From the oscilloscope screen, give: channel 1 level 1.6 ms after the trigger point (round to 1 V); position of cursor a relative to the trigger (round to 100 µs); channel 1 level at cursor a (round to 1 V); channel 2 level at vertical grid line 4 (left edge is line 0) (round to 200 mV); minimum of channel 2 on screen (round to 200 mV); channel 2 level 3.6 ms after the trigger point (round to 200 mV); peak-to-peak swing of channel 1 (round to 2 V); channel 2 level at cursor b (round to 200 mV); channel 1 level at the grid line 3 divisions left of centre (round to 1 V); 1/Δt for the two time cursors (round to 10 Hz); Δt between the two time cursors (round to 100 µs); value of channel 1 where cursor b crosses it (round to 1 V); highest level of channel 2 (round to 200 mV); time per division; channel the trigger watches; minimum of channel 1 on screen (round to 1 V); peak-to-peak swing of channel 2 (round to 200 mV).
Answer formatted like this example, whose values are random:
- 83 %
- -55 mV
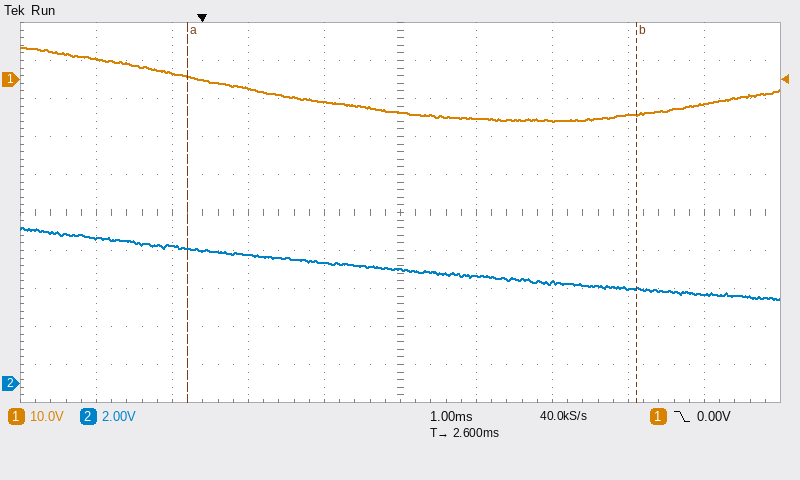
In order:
- -6 V
- -200 µs
- 1 V
- 6.4 V
- 4.4 V
- 5.6 V
- 20 V
- 5.0 V
- 2 V
- 170 Hz
- 5.9 ms
- -9 V
- 8.2 V
- 1 ms
- channel 1
- -11 V
- 3.8 V
